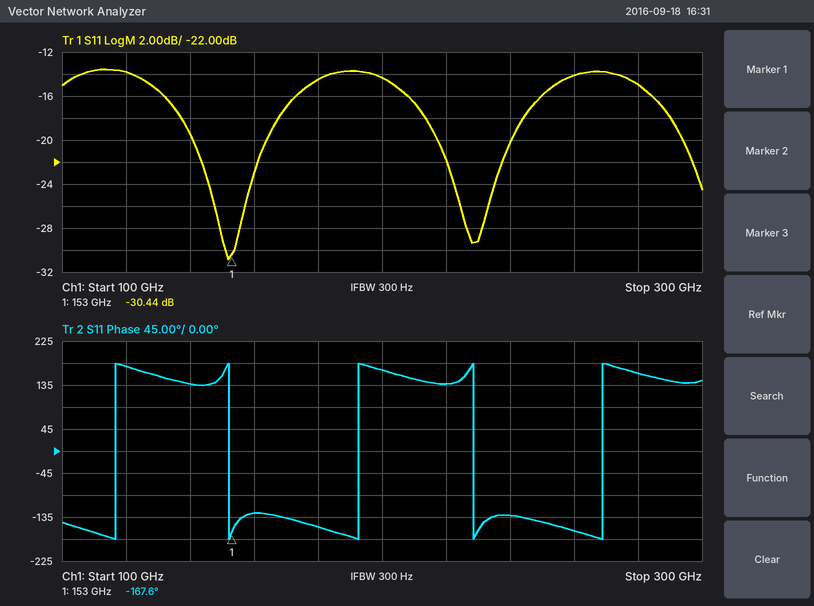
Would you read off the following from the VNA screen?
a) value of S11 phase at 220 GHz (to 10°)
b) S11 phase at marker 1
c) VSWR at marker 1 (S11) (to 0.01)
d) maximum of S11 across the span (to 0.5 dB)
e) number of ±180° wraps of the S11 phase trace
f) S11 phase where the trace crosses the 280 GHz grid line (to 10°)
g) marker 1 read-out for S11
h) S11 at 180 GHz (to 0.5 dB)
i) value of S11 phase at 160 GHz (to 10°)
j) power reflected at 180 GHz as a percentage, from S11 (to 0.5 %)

140°
-167.6°
1.06
-13.5 dB
5
160°
-30.44 dB
-14.5 dB
-130°
3.5 %
